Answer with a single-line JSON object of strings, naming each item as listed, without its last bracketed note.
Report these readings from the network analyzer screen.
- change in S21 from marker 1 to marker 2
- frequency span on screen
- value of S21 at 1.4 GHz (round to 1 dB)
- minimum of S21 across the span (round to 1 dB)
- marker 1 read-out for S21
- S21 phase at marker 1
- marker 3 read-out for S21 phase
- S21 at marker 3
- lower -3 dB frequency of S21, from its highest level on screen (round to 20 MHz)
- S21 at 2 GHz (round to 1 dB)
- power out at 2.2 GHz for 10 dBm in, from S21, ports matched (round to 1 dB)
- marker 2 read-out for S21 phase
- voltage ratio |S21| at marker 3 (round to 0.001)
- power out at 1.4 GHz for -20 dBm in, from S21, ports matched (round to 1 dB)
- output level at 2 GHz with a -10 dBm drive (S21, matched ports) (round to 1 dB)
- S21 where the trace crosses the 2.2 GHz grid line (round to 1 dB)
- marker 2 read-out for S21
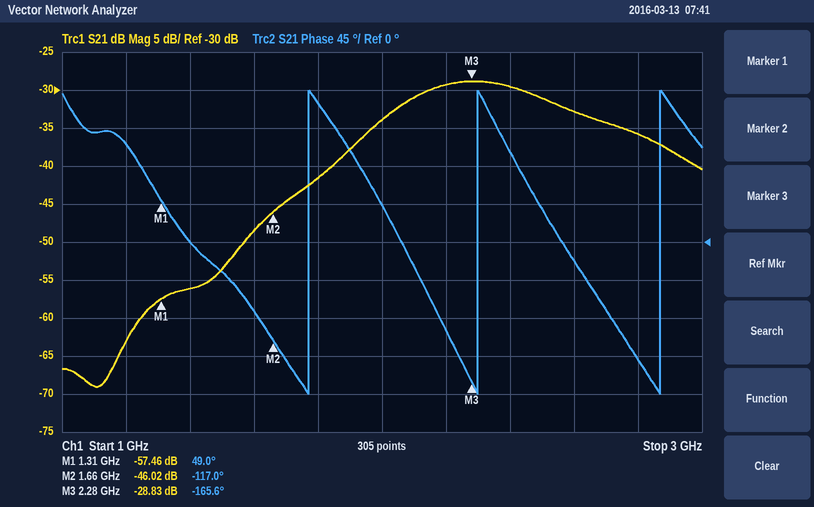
{"change in S21 from marker 1 to marker 2": "11.44 dB", "frequency span on screen": "2 GHz", "value of S21 at 1.4 GHz": "-56 dB", "minimum of S21 across the span": "-69 dB", "marker 1 read-out for S21": "-57.46 dB", "S21 phase at marker 1": "49.0°", "marker 3 read-out for S21 phase": "-165.6°", "S21 at marker 3": "-28.83 dB", "lower -3 dB frequency of S21, from its highest level on screen": "2.06 GHz", "S21 at 2 GHz": "-34 dB", "power out at 2.2 GHz for 10 dBm in, from S21, ports matched": "-19 dBm", "marker 2 read-out for S21 phase": "-117.0°", "voltage ratio |S21| at marker 3": "0.036", "power out at 1.4 GHz for -20 dBm in, from S21, ports matched": "-76 dBm", "output level at 2 GHz with a -10 dBm drive (S21, matched ports)": "-44 dBm", "S21 where the trace crosses the 2.2 GHz grid line": "-29 dB", "marker 2 read-out for S21": "-46.02 dB"}
